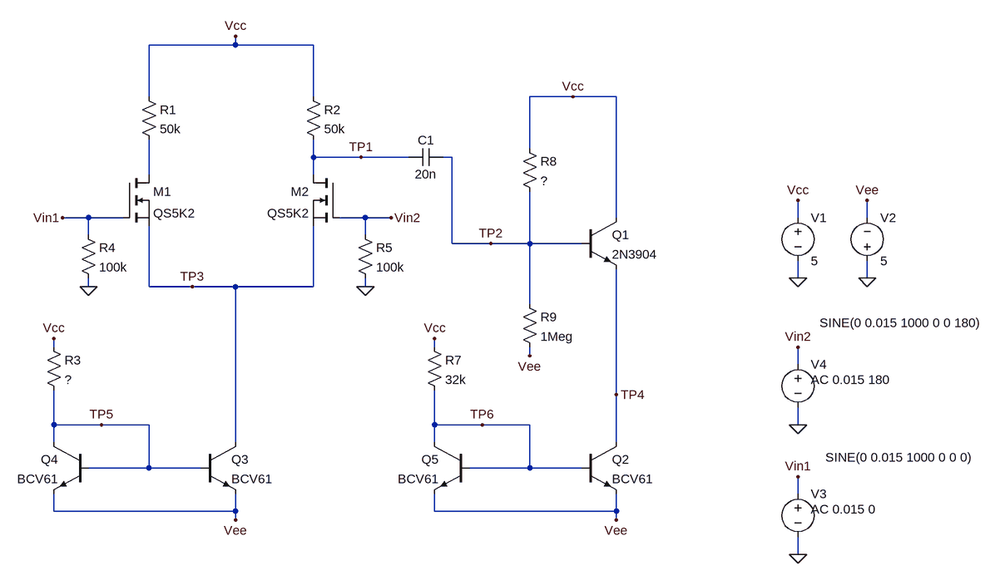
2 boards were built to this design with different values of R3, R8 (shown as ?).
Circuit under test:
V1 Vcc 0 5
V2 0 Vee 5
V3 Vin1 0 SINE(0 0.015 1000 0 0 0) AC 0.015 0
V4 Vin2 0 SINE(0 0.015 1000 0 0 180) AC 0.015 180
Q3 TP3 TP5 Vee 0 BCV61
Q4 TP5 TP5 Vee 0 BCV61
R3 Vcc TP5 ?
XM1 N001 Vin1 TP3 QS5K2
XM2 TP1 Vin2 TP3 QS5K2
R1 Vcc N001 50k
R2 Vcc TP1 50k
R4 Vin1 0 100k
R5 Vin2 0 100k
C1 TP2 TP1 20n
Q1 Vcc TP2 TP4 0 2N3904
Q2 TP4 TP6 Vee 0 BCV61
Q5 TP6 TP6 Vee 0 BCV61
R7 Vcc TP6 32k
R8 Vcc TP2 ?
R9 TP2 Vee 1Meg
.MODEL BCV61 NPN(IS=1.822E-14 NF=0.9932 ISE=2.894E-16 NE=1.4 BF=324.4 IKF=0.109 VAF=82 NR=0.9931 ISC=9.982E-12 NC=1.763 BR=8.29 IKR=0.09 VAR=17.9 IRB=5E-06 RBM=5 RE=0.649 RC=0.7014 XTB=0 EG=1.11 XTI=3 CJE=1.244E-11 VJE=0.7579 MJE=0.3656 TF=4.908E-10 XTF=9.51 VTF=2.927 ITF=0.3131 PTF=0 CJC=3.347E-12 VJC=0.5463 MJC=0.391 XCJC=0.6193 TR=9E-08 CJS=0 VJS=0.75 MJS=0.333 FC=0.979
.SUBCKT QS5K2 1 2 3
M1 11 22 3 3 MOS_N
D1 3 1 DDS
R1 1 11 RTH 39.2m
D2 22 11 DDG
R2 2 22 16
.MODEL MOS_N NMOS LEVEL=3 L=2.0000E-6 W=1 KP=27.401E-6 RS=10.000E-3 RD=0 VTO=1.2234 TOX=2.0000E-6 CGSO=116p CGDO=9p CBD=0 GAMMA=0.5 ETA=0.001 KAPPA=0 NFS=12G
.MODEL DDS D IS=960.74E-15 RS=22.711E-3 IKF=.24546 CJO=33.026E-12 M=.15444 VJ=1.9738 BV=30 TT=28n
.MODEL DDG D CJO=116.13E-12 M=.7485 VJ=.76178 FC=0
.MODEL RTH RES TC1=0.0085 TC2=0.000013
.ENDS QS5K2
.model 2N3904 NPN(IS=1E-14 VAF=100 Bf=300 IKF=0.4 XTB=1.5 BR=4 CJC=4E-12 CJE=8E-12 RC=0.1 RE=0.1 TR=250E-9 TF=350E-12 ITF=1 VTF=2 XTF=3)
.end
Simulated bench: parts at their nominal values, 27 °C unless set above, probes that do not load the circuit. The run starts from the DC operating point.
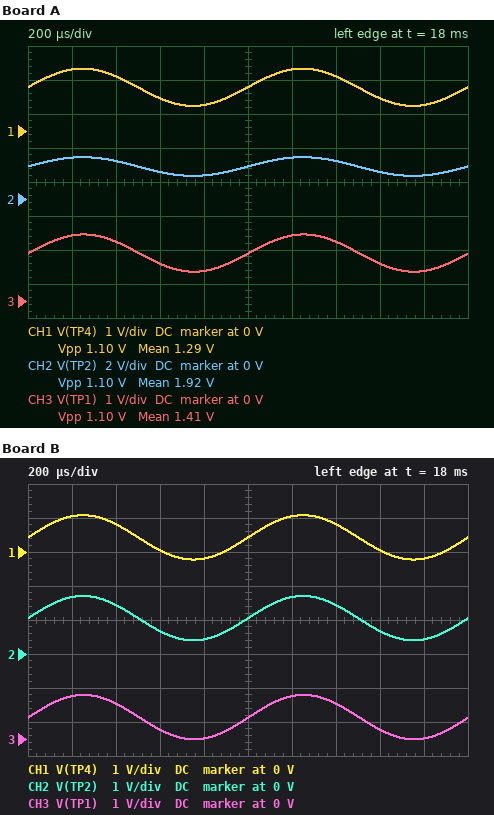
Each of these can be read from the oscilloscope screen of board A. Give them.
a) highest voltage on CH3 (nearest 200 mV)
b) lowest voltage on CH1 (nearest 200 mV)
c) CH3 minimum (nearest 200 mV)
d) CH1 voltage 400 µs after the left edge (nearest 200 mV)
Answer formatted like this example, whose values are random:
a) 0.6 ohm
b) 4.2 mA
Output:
a) 2.0 V
b) 800 mV
c) 800 mV
d) 1.6 V
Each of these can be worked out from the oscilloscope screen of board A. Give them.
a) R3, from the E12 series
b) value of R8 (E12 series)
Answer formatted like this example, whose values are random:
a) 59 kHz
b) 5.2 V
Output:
a) 68 kΩ
b) 390 kΩ
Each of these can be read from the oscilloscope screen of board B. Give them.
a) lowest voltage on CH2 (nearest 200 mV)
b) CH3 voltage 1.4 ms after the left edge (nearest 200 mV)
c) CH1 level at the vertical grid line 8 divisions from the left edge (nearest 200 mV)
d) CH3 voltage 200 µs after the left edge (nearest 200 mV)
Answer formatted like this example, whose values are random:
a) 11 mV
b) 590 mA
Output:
a) 400 mV
b) 1.0 V
c) 0 V
d) 1.2 V
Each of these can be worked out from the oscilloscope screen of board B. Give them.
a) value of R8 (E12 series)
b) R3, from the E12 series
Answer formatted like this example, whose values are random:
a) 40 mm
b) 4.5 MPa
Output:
a) 560 kΩ
b) 56 kΩ
